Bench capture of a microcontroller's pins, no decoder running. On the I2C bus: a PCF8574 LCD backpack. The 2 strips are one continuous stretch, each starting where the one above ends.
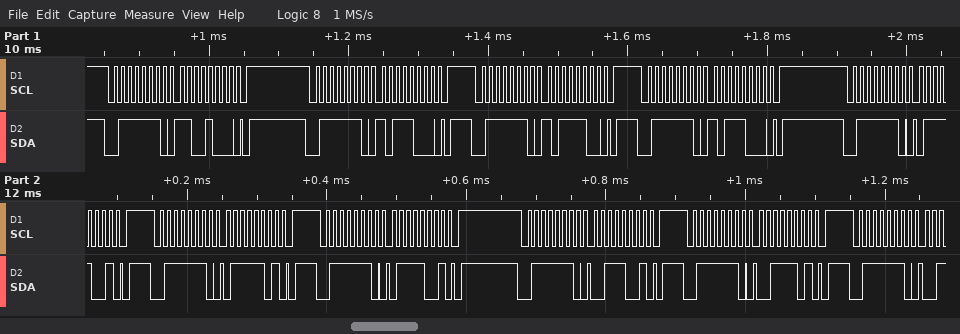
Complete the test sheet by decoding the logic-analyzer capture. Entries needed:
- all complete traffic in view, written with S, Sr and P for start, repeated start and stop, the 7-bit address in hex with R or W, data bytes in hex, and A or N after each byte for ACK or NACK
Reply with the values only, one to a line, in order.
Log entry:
S 3FW A C8 A P S 3FW A B8 A P S 3FW A BC A P S 3FW A B8 A P S 3FW A 79 A P S 3FW A 7D A P S 3FW A 79 A P S 3FW A 39 A P S 3FW A 3D A P S 3FW A
